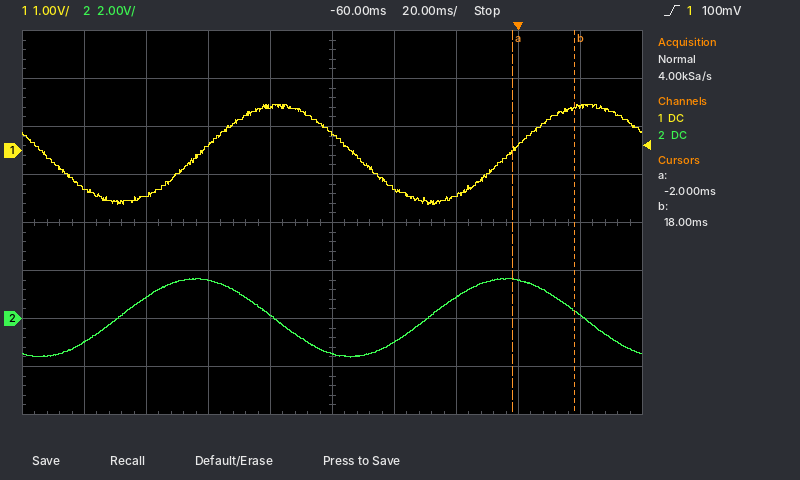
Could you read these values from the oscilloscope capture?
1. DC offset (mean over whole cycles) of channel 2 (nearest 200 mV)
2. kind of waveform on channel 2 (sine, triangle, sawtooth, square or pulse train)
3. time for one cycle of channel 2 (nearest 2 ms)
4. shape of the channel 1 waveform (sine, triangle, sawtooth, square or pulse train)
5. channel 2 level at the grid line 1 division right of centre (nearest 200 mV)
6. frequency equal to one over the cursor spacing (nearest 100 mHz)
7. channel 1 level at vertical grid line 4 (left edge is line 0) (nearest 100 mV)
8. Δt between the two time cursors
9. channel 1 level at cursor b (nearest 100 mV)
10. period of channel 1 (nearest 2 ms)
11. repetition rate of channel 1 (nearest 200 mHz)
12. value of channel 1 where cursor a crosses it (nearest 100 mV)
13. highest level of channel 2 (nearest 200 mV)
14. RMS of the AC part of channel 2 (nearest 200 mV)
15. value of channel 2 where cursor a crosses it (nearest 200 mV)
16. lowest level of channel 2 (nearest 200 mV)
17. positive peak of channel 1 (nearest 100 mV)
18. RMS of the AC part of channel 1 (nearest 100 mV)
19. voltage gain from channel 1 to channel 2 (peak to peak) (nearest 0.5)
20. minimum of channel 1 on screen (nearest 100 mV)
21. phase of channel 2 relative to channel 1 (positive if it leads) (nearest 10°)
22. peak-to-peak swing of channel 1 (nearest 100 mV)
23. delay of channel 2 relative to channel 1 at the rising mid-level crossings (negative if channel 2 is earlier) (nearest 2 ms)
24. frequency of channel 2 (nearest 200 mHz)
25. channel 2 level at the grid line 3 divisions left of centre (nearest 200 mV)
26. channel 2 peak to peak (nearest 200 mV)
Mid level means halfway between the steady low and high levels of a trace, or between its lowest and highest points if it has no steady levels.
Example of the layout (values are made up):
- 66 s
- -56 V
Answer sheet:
- 0.0 V
- sine
- 100 ms
- sine
- -1.0 V
- 50.0 Hz
- 900 mV
- 20 ms
- 900 mV
- 100 ms
- 10.0 Hz
- 0.0 V
- 1.6 V
- 1.2 V
- 1.6 V
- -1.6 V
- 1.0 V
- 700 mV
- 1.5
- -1.1 V
- +90°
- 2.1 V
- -26 ms
- 10.0 Hz
- 800 mV
- 3.2 V
